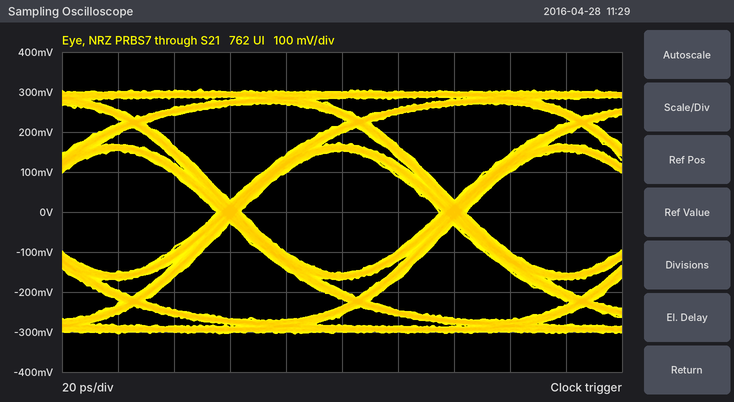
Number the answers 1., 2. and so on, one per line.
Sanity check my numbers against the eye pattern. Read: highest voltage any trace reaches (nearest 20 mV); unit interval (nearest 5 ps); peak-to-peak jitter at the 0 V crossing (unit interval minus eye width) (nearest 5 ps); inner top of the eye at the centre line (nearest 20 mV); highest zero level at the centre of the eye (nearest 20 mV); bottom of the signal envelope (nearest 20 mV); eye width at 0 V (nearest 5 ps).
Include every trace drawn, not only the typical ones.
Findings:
1. 300 mV
2. 80 ps
3. 10 ps
4. 160 mV
5. -160 mV
6. -300 mV
7. 70 ps
